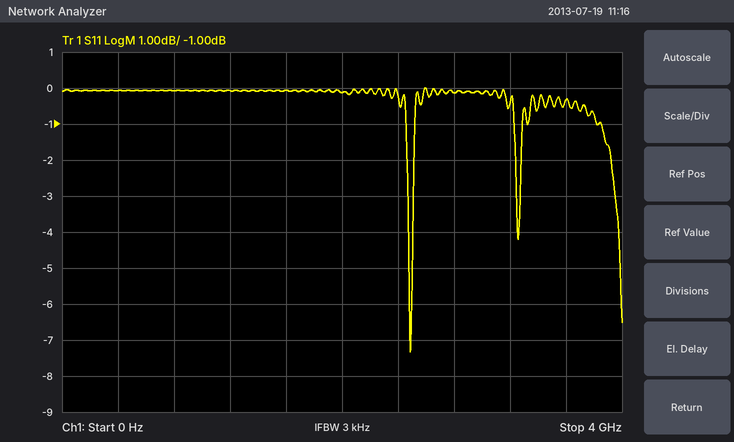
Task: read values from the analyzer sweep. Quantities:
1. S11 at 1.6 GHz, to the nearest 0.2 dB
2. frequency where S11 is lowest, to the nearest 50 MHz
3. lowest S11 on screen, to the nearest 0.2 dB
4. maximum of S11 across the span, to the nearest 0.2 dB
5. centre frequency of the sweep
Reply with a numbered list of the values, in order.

1. 0.0 dB
2. 2.50 GHz
3. -7.4 dB
4. 0.0 dB
5. 2 GHz
